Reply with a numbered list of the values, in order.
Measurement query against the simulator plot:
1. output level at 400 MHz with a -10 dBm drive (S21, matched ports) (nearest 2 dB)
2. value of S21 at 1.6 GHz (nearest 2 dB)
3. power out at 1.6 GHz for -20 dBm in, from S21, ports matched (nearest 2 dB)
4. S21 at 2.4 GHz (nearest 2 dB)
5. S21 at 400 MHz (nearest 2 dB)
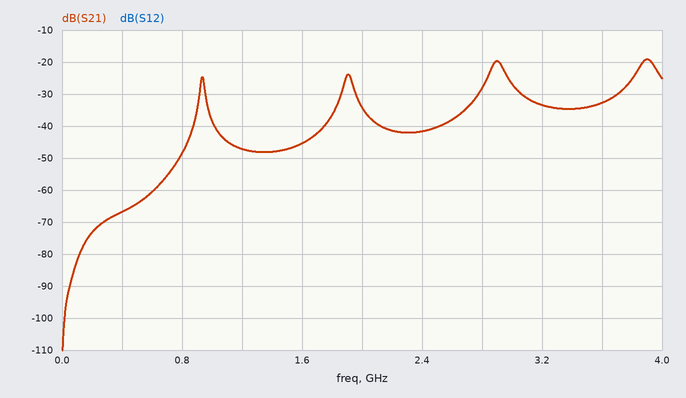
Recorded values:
1. -76 dBm
2. -46 dB
3. -66 dBm
4. -42 dB
5. -66 dB
